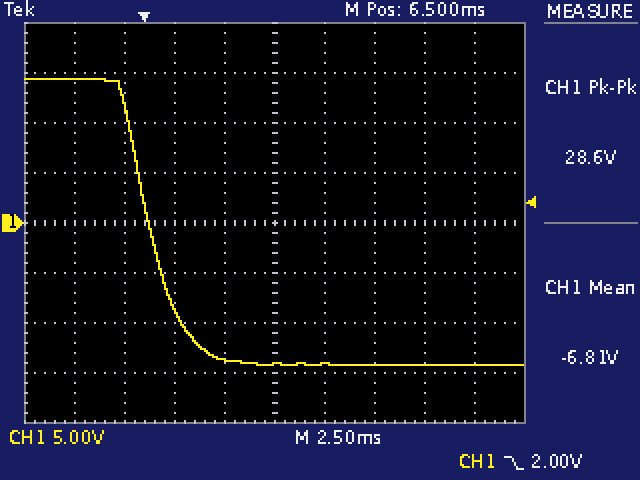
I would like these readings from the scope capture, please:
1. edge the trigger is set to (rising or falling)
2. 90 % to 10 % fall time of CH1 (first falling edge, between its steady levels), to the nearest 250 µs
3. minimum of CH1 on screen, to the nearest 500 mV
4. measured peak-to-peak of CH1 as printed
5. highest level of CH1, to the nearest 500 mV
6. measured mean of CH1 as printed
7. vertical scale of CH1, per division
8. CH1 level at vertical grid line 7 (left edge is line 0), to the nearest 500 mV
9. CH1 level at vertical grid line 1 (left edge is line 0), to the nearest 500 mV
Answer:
falling
3.25 ms
-14.0 V
28.6 V
14.5 V
-6.81 V
5 V
-14.0 V
14.5 V
